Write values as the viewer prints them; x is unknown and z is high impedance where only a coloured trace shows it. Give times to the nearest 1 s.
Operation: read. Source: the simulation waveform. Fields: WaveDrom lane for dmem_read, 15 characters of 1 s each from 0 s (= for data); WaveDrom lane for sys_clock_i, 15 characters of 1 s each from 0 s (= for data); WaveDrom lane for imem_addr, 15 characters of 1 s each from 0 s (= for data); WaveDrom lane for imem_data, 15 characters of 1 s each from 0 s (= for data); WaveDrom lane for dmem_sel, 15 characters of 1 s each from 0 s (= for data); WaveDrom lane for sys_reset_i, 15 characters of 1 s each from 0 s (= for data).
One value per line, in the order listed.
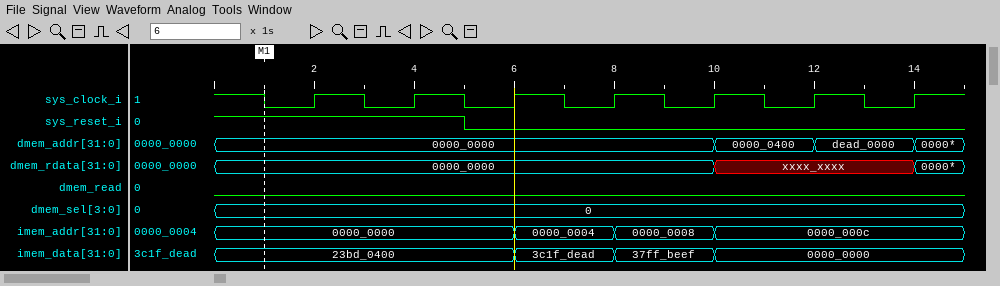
{name: 'dmem_read', wave: '0..............'}
{name: 'sys_clock_i', wave: '101010101010101'}
{name: 'imem_addr', wave: '=.....=.=.=....', data: '0000_0000 0000_0004 0000_0008 0000_000c'}
{name: 'imem_data', wave: '=.....=.=.=....', data: '23bd_0400 3c1f_dead 37ff_beef 0000_0000'}
{name: 'dmem_sel', wave: '=..............', data: '0'}
{name: 'sys_reset_i', wave: '1....0.........'}
